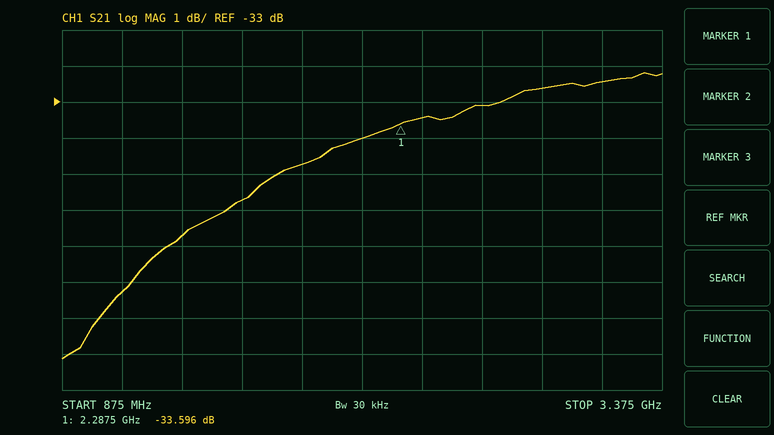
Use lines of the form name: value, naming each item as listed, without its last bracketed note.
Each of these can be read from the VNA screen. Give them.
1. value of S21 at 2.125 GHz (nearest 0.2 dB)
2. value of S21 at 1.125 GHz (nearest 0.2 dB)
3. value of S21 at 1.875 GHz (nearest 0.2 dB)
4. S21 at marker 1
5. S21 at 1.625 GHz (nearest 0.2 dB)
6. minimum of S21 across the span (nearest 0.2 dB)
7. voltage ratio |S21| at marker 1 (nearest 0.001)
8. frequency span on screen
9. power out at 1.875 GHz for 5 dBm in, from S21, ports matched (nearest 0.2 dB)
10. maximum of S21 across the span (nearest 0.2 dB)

value of S21 at 2.125 GHz: -34.0 dB
value of S21 at 1.125 GHz: -38.2 dB
value of S21 at 1.875 GHz: -34.8 dB
S21 at marker 1: -33.596 dB
S21 at 1.625 GHz: -35.8 dB
minimum of S21 across the span: -40.2 dB
voltage ratio |S21| at marker 1: 0.021
frequency span on screen: 2.5 GHz
power out at 1.875 GHz for 5 dBm in, from S21, ports matched: -29.8 dBm
maximum of S21 across the span: -32.2 dB
